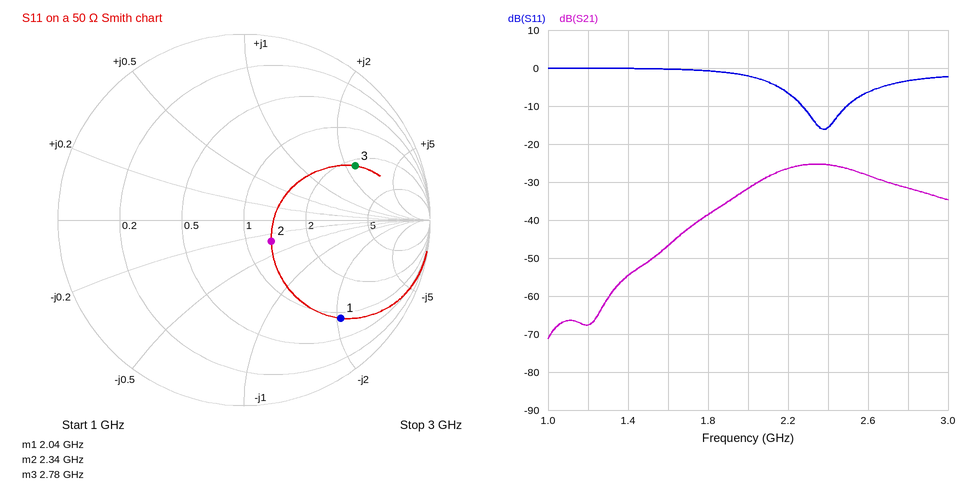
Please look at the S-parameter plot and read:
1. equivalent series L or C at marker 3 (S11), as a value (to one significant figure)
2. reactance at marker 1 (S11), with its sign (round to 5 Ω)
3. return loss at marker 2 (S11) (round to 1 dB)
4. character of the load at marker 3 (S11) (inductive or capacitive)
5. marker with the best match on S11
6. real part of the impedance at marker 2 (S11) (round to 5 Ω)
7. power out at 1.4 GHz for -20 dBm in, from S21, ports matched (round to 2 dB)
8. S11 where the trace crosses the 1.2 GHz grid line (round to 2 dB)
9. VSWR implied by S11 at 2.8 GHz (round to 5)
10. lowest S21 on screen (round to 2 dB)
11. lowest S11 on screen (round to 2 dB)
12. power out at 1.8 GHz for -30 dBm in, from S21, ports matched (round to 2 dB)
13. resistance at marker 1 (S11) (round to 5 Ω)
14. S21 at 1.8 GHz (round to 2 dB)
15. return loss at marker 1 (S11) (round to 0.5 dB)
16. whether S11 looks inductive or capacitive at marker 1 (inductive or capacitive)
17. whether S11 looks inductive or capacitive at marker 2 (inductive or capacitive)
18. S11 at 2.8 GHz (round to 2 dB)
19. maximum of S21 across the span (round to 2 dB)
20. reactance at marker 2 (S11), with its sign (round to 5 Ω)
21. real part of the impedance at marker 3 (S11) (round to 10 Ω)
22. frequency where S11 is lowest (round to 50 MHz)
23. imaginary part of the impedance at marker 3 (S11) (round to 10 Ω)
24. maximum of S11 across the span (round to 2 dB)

7 nH
-105 Ω
15 dB
inductive
marker 2
65 Ω
-74 dBm
0 dB
5
-72 dB
-16 dB
-68 dBm
45 Ω
-38 dB
2.5 dB
capacitive
capacitive
-4 dB
-26 dB
-15 Ω
110 Ω
2.40 GHz
+120 Ω
0 dB
